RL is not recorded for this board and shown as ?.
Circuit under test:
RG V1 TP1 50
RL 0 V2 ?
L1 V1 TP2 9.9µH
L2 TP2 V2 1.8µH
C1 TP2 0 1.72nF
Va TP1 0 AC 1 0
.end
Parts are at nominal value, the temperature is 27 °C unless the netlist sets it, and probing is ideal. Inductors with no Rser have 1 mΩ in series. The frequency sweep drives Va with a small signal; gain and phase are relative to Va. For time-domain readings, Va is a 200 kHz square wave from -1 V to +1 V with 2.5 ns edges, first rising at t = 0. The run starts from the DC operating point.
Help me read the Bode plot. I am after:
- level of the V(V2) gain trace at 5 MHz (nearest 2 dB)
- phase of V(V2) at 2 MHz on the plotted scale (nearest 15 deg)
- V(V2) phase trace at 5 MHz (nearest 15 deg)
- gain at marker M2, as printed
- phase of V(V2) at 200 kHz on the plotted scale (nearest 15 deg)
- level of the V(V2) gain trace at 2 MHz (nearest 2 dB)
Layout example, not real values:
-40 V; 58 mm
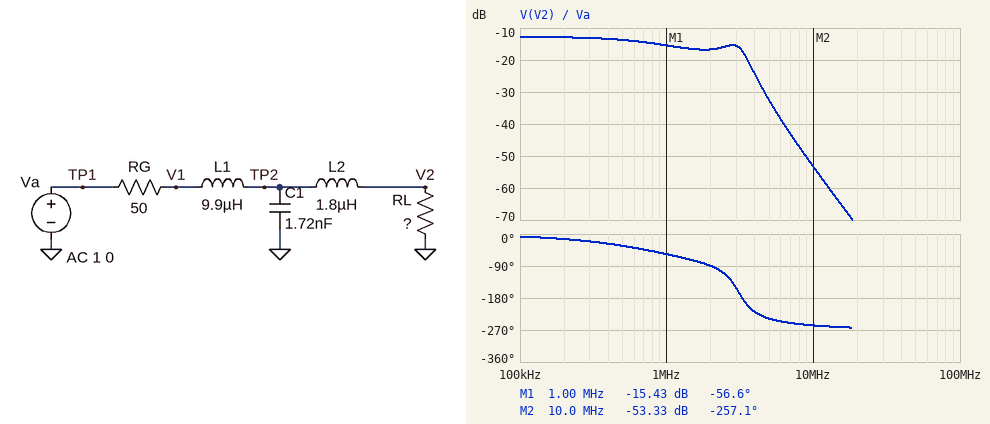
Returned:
-32 dB; -90 deg; -240 deg; -53.33 dB; -15 deg; -16 dB
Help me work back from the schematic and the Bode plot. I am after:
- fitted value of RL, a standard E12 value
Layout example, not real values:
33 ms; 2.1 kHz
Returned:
15 Ω
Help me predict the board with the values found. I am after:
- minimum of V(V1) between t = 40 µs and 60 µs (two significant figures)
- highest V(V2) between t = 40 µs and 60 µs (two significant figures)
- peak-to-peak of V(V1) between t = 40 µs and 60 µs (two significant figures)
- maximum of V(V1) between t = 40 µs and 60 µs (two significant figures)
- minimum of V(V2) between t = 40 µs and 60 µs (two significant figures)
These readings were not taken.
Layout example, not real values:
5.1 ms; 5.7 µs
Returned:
-1.8 V; 230 mV; 3.5 V; 1.8 V; -230 mV
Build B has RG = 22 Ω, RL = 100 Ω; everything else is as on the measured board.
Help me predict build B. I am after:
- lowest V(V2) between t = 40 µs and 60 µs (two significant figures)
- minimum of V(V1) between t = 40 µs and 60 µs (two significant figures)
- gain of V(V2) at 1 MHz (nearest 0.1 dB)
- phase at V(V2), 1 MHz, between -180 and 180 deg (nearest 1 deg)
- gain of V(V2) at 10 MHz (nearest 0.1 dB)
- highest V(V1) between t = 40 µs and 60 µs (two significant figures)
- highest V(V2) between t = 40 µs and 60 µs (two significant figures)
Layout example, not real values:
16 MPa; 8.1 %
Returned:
-1.1 V; -1.2 V; -0.3 dB; -60 deg; -39.6 dB; 1.2 V; 1.1 V
